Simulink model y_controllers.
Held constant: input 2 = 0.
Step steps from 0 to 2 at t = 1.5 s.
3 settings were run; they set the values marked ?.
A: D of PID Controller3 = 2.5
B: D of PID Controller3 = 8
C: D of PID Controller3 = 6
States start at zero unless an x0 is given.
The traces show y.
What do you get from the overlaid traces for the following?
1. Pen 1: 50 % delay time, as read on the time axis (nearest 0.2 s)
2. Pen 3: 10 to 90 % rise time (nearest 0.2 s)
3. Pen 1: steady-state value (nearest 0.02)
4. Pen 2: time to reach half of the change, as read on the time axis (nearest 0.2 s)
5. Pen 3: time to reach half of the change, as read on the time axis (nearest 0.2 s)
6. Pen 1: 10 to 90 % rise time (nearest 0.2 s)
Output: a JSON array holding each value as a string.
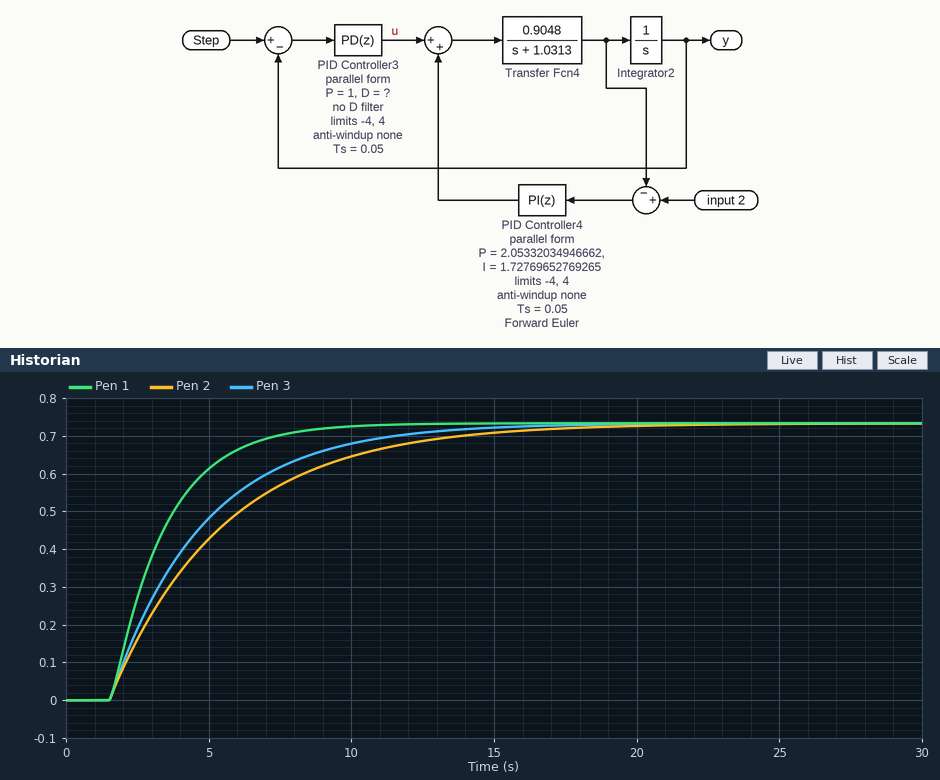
["3.0 s", "7.2 s", "0.74", "4.2 s", "3.8 s", "4.2 s"]
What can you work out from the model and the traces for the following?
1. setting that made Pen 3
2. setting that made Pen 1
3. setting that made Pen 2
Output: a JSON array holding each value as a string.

["C", "A", "B"]
